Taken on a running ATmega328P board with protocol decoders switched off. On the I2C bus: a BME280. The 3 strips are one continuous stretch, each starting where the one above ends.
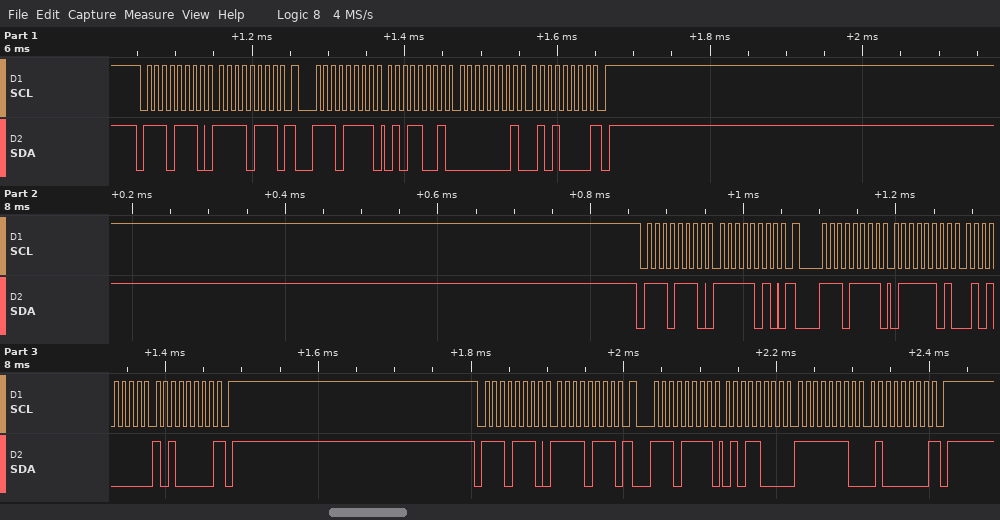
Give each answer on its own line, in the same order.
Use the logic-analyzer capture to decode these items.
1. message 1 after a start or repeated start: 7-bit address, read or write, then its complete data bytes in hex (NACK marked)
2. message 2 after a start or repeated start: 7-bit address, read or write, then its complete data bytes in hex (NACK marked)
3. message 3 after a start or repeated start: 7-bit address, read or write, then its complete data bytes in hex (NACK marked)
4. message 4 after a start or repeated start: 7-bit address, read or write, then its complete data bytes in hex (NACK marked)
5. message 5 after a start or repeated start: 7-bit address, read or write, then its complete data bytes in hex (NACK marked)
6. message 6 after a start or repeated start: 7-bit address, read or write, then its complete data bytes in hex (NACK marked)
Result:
0x77 write: F7
0x77 read: 59 01 50 NACK
0x77 write: FA
0x77 read: 7D 50 A0 NACK
0x77 write: F7
0x77 read: 58 FE 40 NACK
